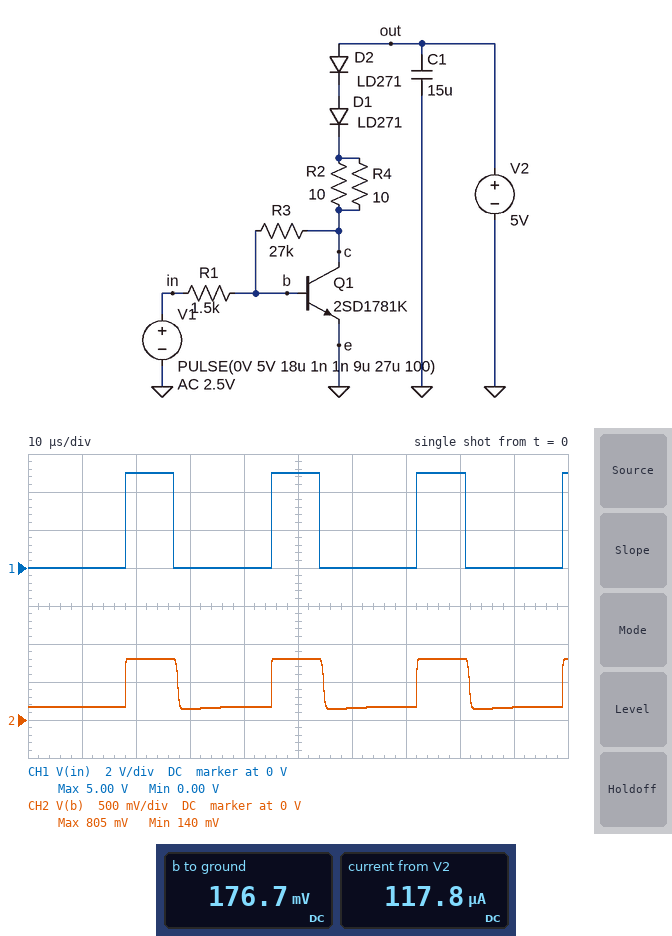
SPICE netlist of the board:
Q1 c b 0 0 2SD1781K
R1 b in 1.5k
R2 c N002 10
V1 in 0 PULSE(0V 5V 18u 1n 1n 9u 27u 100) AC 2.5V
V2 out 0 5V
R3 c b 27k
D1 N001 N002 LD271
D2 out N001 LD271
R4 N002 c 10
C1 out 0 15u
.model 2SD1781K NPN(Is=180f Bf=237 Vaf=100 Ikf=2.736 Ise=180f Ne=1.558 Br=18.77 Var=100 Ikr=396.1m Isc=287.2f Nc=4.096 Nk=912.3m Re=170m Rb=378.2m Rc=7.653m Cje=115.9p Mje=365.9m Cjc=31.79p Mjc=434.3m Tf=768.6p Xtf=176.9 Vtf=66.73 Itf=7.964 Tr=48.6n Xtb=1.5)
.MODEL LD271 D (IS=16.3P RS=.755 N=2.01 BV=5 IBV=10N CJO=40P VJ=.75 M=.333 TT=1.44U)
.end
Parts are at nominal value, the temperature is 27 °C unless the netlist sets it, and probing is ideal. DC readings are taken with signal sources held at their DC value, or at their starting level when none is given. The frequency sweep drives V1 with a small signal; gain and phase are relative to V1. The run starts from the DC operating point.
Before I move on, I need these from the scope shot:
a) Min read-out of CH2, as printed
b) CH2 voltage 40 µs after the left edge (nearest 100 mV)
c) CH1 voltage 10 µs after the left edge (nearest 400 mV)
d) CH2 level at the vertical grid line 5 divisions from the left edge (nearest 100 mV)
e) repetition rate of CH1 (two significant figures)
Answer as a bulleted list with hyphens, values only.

- 140 mV
- 200 mV
- 0 V
- 800 mV
- 37 kHz
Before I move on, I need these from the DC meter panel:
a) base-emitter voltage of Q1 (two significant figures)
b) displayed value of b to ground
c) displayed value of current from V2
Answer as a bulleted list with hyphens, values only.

- 180 mV
- 176.7 mV
- 117.8 µA
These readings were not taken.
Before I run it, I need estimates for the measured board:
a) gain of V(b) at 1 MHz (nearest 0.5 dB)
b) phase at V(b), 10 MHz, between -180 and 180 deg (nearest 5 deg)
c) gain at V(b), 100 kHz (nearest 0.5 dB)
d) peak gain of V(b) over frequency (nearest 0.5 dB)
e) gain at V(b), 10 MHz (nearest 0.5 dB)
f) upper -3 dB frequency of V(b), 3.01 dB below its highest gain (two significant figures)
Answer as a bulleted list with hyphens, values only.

- -4.5 dB
- -85 deg
- -0.5 dB
- -0.5 dB
- -22.5 dB
- 780 kHz
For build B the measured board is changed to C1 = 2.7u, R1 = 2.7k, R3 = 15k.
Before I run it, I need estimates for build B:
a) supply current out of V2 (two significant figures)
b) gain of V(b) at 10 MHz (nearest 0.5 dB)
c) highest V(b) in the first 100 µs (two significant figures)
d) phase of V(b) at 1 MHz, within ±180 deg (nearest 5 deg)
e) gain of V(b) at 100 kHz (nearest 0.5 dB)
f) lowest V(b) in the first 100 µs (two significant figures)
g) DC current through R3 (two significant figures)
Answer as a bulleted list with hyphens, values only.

- 230 µA
- -30.0 dB
- 780 mV
- -70 deg
- -2.5 dB
- 410 mV
- 190 µA
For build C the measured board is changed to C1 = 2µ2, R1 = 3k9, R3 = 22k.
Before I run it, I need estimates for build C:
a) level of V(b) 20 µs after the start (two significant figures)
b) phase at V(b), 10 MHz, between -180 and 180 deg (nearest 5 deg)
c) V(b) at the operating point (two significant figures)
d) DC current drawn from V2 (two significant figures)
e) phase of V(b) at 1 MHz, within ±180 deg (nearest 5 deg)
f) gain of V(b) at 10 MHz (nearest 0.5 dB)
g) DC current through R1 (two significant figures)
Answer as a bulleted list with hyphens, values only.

- 760 mV
- -90 deg
- 500 mV
- 170 µA
- -75 deg
- -33.0 dB
- 130 µA
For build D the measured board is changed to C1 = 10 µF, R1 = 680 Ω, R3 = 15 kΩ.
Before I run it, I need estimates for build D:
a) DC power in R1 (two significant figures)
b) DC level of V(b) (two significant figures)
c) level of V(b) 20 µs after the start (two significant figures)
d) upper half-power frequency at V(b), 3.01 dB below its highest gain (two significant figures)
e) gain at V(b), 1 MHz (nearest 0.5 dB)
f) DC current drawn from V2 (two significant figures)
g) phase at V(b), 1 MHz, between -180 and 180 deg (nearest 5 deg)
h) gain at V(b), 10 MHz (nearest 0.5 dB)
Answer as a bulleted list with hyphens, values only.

- 30 µW
- 140 mV
- 820 mV
- 1.7 MHz
- -1.5 dB
- 210 µA
- -30 deg
- -15.5 dB
